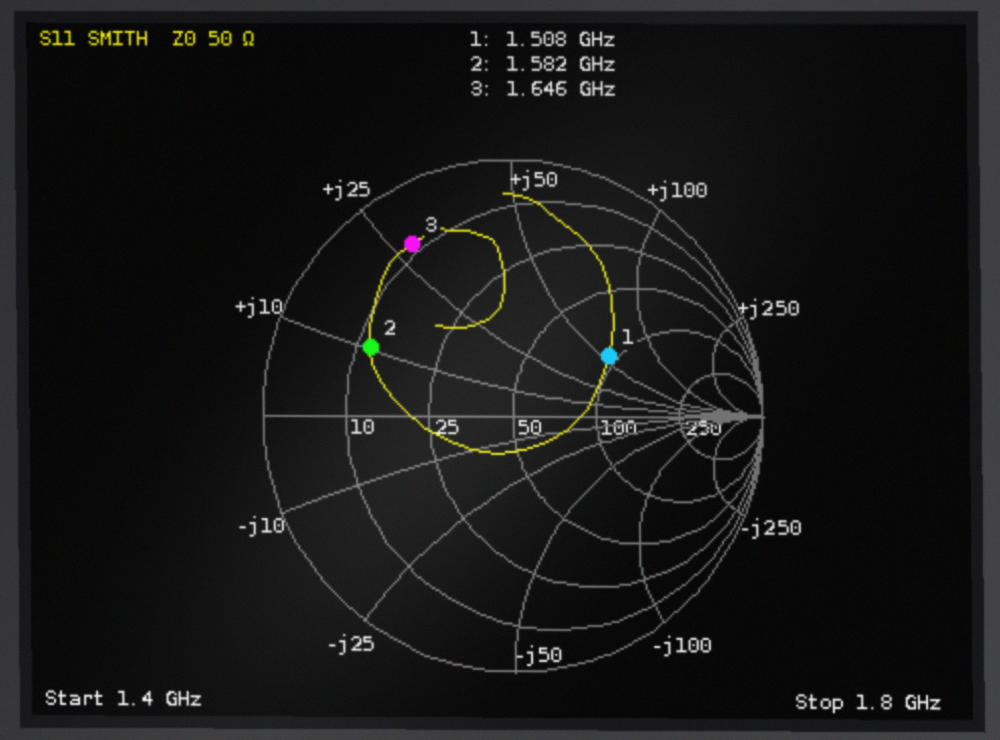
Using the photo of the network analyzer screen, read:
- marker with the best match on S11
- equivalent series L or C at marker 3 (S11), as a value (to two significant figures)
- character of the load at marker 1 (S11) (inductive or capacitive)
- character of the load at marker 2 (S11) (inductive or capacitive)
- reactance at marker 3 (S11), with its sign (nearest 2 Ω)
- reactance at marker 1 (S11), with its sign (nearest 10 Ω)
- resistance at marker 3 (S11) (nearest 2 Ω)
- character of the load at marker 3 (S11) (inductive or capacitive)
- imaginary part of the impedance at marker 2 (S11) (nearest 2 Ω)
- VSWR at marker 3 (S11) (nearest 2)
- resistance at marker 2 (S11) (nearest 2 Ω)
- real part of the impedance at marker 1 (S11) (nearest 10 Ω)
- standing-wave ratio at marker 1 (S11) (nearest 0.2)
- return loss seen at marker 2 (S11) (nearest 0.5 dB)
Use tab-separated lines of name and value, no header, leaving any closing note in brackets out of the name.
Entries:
marker with the best match on S11	marker 1
equivalent series L or C at marker 3 (S11), as a value	2.7 nH
character of the load at marker 1 (S11)	inductive
character of the load at marker 2 (S11)	inductive
reactance at marker 3 (S11), with its sign	+28 Ω
reactance at marker 1 (S11), with its sign	+50 Ω
resistance at marker 3 (S11)	8 Ω
character of the load at marker 3 (S11)	inductive
imaginary part of the impedance at marker 2 (S11)	+10 Ω
VSWR at marker 3 (S11)	8
resistance at marker 2 (S11)	12 Ω
real part of the impedance at marker 1 (S11)	90 Ω
standing-wave ratio at marker 1 (S11)	2.6
return loss seen at marker 2 (S11)	4.0 dB
